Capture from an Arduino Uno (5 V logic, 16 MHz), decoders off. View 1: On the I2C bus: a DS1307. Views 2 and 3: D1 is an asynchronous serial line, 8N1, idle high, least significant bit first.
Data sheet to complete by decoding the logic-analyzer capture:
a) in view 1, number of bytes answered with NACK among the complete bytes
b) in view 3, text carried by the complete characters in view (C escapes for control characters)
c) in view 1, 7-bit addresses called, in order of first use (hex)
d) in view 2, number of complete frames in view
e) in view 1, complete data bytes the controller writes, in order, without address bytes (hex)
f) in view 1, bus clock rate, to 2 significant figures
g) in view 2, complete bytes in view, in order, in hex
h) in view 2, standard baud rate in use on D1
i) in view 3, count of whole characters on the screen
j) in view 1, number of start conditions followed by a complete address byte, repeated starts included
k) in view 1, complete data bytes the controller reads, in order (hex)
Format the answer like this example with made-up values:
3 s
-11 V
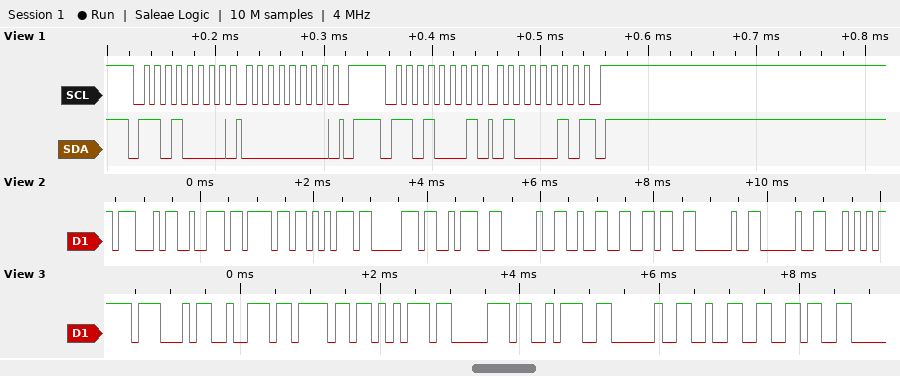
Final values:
1
"Group: 26"
0x68
12
00
100 kHz
47 72 6F 75 70 3A 20 32 36 20 20 54
9600 baud
9
2
42
